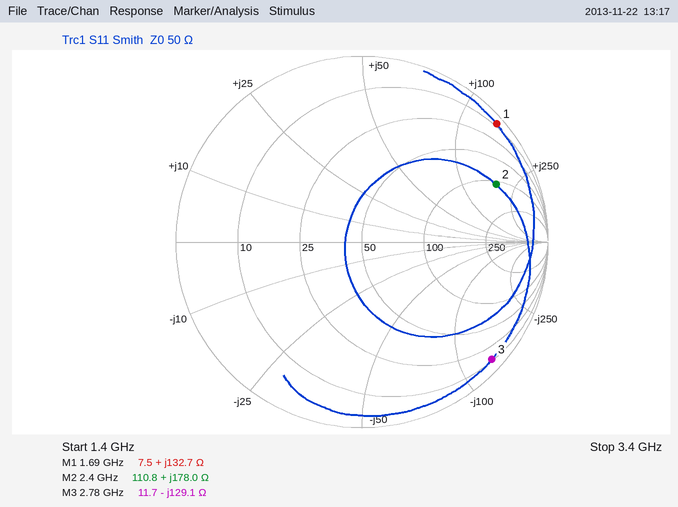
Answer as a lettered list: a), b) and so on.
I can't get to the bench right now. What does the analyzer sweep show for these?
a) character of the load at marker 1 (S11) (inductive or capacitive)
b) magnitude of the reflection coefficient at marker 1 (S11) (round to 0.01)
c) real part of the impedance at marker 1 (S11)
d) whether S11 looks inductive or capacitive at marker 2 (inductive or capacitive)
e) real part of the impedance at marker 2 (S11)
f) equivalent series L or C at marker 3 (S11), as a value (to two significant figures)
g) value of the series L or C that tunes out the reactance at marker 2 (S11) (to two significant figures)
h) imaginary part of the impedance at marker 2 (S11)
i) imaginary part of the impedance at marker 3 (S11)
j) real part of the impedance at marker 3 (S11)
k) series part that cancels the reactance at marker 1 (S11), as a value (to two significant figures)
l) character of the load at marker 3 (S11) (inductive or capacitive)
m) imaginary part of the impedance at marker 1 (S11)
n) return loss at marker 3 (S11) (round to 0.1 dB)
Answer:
a) inductive
b) 0.96
c) 7.5 Ω
d) inductive
e) 110.8 Ω
f) 440 fF
g) 370 fF
h) +178.0 Ω
i) -129.1 Ω
j) 11.7 Ω
k) 710 fF
l) capacitive
m) +132.7 Ω
n) 0.5 dB
